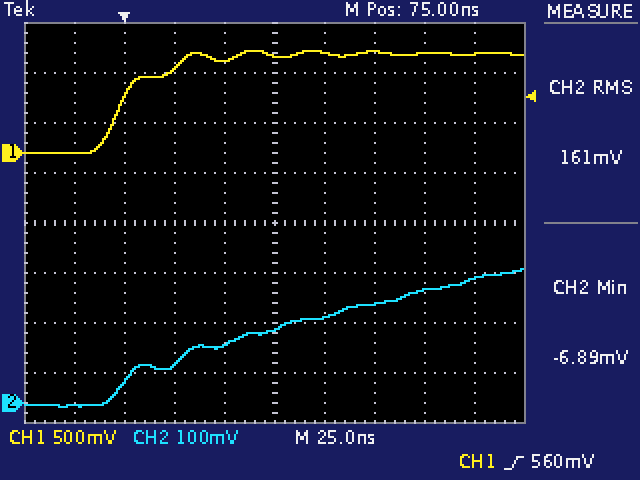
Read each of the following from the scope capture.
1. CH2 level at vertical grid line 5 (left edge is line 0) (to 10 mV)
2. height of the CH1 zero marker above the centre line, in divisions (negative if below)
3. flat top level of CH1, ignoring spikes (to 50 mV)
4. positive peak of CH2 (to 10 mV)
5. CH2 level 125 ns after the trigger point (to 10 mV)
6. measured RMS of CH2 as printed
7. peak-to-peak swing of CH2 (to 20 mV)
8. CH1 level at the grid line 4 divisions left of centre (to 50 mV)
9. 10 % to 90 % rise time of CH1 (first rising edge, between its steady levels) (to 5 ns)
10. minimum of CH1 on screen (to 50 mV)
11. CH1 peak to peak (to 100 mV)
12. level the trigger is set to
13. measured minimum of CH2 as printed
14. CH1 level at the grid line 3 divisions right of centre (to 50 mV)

150 mV
+1.4 div
1.00 V
270 mV
200 mV
161 mV
280 mV
0 mV
40 ns
0 mV
1.00 V
560 mV
-6.89 mV
1.00 V
